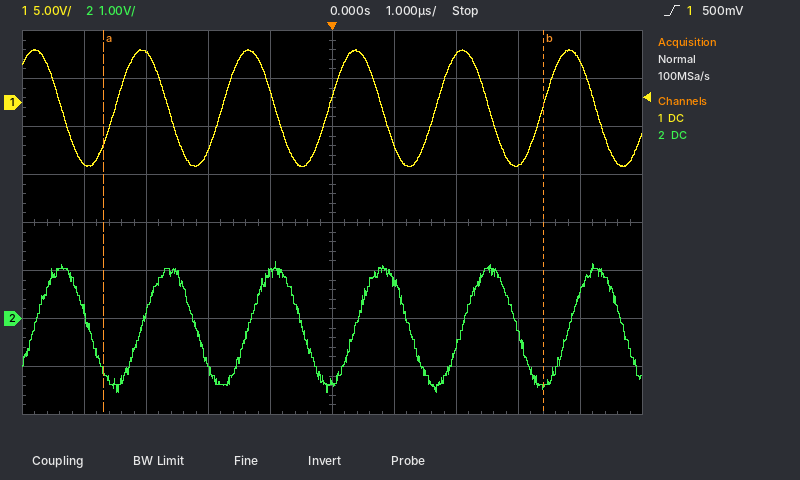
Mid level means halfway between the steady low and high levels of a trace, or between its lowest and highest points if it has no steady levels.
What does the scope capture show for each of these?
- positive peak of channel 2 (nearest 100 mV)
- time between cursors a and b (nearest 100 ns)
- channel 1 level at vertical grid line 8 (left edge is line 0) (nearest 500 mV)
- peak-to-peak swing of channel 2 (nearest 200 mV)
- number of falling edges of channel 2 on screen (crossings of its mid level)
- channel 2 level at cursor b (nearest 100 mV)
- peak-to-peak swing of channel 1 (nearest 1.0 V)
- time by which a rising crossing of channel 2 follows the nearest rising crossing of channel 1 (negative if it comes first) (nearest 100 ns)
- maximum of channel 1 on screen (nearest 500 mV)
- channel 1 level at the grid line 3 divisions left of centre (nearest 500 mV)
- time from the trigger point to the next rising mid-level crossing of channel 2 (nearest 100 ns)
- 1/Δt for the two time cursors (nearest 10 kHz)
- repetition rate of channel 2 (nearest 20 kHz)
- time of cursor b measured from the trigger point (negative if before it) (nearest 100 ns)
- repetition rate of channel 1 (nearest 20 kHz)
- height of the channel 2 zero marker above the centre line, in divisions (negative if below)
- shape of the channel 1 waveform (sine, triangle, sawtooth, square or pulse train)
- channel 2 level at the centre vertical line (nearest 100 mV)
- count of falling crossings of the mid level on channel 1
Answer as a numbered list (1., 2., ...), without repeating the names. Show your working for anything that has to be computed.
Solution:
1. 1.2 V
2. 7.1 µs
3. -6.5 V
4. 2.8 V
5. 6
6. -1.4 V
7. 12.0 V
8. +400 ns
9. 5.5 V
10. 5.0 V
11. 400 ns
12. 1 / 7.1 µs ≈ 140 kHz
13. 580 kHz
14. +3.4 µs
15. 580 kHz
16. -2.0 div
17. sine
18. -1.3 V
19. 6
